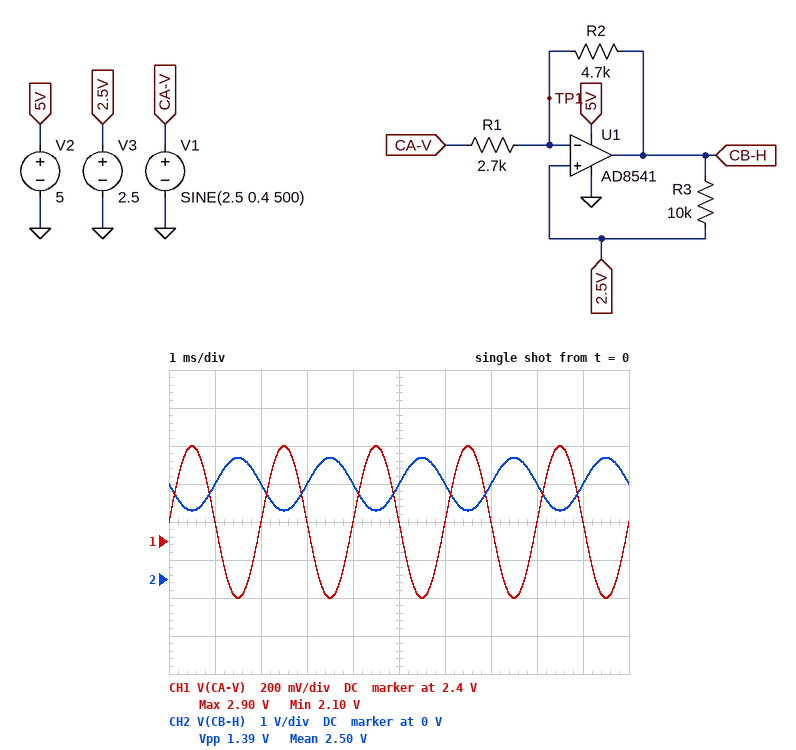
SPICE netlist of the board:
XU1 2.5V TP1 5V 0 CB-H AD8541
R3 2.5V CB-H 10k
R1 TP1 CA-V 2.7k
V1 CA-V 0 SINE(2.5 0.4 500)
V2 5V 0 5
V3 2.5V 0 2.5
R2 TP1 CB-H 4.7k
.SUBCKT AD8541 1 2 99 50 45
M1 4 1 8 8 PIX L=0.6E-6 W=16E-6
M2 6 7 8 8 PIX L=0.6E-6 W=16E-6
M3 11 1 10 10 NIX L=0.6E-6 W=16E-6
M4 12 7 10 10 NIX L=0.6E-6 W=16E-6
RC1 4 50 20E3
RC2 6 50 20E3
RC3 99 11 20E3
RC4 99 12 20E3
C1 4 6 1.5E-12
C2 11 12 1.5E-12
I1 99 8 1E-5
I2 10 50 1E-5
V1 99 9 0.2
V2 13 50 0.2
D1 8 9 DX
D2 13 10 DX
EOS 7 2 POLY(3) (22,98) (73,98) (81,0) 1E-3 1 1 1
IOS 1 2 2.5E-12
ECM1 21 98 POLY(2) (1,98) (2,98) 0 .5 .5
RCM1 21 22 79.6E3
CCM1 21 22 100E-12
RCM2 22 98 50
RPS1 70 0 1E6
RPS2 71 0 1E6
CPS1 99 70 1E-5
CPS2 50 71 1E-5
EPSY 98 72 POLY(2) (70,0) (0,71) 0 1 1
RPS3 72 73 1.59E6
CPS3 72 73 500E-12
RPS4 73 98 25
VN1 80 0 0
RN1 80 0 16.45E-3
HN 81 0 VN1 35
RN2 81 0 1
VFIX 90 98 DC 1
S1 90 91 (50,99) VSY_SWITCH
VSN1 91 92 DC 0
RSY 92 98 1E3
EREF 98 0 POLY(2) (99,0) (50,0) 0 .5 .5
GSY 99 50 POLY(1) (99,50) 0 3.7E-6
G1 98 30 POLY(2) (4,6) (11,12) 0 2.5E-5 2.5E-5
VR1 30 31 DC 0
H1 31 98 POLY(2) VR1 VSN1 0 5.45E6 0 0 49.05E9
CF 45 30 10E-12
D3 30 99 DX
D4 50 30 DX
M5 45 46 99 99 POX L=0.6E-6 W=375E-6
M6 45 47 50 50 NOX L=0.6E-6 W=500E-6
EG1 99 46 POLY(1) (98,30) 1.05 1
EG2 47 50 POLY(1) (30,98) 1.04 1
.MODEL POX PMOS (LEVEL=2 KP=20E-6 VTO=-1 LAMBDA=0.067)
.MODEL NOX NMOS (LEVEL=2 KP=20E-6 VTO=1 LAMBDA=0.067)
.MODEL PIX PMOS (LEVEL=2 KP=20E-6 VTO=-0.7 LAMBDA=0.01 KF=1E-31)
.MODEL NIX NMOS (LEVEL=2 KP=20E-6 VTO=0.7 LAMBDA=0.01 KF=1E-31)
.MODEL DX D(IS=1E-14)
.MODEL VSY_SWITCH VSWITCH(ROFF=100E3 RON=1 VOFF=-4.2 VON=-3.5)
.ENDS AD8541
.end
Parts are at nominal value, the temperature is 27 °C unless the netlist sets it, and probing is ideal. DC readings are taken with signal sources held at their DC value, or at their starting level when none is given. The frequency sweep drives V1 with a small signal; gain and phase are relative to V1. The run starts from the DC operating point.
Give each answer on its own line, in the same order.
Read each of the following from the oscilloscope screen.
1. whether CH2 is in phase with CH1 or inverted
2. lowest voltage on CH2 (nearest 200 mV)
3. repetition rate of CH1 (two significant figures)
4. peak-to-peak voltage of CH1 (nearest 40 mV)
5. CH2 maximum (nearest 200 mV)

inverted
1.8 V
500 Hz
800 mV
3.2 V
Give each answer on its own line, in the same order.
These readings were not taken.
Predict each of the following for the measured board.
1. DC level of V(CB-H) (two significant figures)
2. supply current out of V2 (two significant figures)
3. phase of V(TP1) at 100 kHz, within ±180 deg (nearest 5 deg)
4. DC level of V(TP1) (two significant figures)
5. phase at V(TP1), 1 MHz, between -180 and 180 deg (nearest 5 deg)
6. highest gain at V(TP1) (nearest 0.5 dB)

2.5 V
56 µA
75 deg
2.5 V
20 deg
-2.5 dB
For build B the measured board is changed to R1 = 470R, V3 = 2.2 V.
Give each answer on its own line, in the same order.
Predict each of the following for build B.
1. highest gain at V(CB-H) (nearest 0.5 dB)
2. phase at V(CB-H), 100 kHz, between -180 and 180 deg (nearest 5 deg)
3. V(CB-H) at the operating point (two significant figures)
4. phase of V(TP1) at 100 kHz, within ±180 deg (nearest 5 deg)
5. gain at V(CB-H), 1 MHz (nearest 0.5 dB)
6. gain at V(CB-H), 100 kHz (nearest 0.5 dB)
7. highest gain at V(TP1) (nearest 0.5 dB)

-47.0 dB
5 deg
14 mV
0 deg
-50.0 dB
-52.5 dB
-1.0 dB
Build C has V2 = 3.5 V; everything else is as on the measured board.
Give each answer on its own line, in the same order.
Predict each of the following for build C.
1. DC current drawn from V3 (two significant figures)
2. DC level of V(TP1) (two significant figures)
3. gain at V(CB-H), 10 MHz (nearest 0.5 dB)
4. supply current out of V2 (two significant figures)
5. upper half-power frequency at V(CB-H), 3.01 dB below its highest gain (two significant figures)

400 nA
2.5 V
-20.0 dB
49 µA
440 kHz
